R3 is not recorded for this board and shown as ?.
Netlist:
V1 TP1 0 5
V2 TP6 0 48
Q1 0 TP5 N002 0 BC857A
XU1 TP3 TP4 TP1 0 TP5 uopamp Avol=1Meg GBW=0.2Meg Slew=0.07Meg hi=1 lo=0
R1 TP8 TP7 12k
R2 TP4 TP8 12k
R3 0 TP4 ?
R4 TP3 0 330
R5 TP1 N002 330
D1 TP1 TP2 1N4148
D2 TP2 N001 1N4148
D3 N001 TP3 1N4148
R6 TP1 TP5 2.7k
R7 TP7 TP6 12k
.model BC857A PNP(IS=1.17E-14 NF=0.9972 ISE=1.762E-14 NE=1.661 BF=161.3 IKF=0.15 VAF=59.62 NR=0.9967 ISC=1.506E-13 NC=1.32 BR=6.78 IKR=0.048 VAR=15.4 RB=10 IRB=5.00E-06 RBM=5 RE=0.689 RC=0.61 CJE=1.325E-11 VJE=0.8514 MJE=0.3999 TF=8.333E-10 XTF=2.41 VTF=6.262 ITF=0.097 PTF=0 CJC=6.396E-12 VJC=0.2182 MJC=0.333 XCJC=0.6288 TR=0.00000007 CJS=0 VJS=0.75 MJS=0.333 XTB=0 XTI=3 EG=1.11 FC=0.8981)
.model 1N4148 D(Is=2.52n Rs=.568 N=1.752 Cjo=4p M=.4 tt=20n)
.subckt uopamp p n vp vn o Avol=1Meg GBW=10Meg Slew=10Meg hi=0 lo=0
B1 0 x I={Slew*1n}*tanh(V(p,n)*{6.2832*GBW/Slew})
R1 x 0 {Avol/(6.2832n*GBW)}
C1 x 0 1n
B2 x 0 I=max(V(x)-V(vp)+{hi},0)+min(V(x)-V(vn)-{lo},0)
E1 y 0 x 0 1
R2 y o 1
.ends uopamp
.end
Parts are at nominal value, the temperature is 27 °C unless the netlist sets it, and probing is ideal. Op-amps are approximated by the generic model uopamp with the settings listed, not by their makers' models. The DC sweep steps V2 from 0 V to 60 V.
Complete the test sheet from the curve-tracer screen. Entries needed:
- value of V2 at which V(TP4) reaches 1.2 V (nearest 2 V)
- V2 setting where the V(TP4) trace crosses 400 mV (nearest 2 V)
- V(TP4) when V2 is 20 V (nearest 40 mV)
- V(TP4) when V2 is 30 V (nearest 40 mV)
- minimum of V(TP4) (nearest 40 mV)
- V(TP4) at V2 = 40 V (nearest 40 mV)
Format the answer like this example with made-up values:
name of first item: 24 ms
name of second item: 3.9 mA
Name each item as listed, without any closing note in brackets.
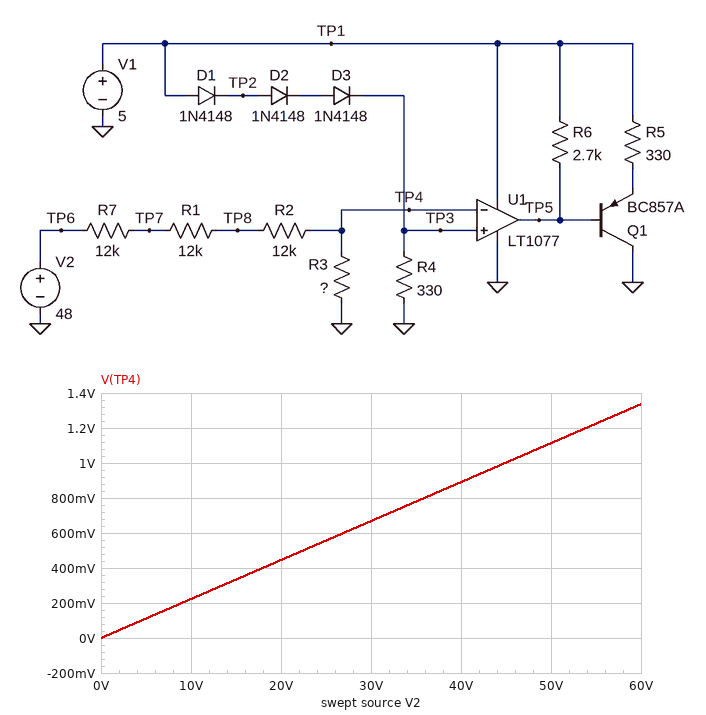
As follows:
value of V2 at which V(TP4) reaches 1.2 V: 54 V
V2 setting where the V(TP4) trace crosses 400 mV: 18 V
V(TP4) when V2 is 20 V: 440 mV
V(TP4) when V2 is 30 V: 680 mV
minimum of V(TP4): 0 V
V(TP4) at V2 = 40 V: 880 mV
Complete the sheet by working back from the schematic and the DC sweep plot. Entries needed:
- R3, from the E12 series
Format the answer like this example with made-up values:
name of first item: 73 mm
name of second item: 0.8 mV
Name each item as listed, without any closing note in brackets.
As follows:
R3, from the E12 series: 820 Ω
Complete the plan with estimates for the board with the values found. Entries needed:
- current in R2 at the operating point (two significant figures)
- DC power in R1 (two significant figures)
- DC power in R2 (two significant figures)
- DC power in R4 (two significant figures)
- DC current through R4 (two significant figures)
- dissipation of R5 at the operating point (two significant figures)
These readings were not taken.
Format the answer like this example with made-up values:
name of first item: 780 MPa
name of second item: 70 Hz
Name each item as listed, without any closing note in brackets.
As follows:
current in R2 at the operating point: 1.3 mA
DC power in R1: 20 mW
DC power in R2: 20 mW
DC power in R4: 26 mW
DC current through R4: 8.9 mA
dissipation of R5 at the operating point: 370 µW
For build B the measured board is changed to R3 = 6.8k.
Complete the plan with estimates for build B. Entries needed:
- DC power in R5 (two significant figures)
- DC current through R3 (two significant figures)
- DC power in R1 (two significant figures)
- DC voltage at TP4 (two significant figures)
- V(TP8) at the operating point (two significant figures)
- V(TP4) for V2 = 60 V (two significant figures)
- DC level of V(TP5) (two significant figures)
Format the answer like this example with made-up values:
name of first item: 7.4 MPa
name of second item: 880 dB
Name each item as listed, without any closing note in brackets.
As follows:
DC power in R5: 55 mW
DC current through R3: 1.1 mA
DC power in R1: 15 mW
DC voltage at TP4: 7.6 V
V(TP8) at the operating point: 21 V
V(TP4) for V2 = 60 V: 9.5 V
DC level of V(TP5): 1.9 mV
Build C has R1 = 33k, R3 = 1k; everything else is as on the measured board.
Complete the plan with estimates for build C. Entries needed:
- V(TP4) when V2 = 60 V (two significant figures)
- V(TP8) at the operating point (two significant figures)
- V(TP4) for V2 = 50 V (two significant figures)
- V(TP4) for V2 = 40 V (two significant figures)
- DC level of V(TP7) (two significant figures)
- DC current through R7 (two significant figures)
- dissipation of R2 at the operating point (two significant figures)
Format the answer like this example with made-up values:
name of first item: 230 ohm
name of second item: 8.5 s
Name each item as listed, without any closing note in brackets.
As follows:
V(TP4) when V2 = 60 V: 1.0 V
V(TP8) at the operating point: 11 V
V(TP4) for V2 = 50 V: 860 mV
V(TP4) for V2 = 40 V: 690 mV
DC level of V(TP7): 38 V
DC current through R7: 830 µA
dissipation of R2 at the operating point: 8.2 mW
